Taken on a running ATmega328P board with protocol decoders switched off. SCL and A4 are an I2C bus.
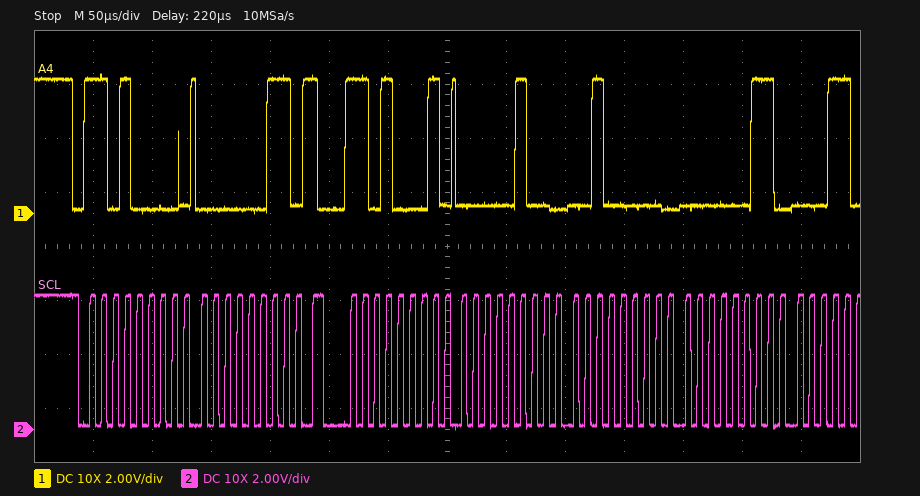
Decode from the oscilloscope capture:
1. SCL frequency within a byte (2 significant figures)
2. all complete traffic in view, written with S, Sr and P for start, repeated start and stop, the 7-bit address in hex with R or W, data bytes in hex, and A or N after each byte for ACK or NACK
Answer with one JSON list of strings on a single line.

["100 kHz", "S 68W A 03 A Sr 68R A 04 A 20 A 03 A"]
